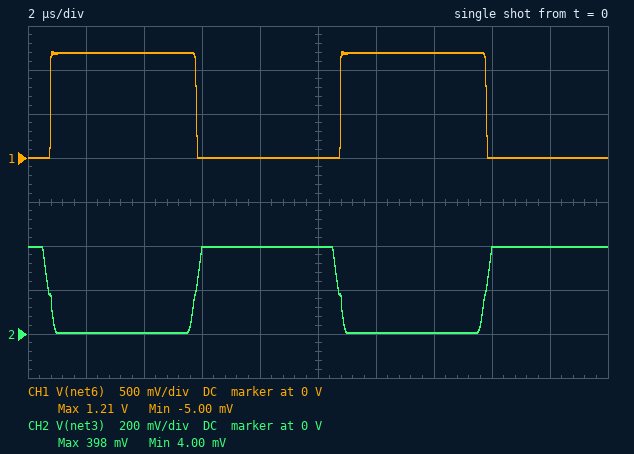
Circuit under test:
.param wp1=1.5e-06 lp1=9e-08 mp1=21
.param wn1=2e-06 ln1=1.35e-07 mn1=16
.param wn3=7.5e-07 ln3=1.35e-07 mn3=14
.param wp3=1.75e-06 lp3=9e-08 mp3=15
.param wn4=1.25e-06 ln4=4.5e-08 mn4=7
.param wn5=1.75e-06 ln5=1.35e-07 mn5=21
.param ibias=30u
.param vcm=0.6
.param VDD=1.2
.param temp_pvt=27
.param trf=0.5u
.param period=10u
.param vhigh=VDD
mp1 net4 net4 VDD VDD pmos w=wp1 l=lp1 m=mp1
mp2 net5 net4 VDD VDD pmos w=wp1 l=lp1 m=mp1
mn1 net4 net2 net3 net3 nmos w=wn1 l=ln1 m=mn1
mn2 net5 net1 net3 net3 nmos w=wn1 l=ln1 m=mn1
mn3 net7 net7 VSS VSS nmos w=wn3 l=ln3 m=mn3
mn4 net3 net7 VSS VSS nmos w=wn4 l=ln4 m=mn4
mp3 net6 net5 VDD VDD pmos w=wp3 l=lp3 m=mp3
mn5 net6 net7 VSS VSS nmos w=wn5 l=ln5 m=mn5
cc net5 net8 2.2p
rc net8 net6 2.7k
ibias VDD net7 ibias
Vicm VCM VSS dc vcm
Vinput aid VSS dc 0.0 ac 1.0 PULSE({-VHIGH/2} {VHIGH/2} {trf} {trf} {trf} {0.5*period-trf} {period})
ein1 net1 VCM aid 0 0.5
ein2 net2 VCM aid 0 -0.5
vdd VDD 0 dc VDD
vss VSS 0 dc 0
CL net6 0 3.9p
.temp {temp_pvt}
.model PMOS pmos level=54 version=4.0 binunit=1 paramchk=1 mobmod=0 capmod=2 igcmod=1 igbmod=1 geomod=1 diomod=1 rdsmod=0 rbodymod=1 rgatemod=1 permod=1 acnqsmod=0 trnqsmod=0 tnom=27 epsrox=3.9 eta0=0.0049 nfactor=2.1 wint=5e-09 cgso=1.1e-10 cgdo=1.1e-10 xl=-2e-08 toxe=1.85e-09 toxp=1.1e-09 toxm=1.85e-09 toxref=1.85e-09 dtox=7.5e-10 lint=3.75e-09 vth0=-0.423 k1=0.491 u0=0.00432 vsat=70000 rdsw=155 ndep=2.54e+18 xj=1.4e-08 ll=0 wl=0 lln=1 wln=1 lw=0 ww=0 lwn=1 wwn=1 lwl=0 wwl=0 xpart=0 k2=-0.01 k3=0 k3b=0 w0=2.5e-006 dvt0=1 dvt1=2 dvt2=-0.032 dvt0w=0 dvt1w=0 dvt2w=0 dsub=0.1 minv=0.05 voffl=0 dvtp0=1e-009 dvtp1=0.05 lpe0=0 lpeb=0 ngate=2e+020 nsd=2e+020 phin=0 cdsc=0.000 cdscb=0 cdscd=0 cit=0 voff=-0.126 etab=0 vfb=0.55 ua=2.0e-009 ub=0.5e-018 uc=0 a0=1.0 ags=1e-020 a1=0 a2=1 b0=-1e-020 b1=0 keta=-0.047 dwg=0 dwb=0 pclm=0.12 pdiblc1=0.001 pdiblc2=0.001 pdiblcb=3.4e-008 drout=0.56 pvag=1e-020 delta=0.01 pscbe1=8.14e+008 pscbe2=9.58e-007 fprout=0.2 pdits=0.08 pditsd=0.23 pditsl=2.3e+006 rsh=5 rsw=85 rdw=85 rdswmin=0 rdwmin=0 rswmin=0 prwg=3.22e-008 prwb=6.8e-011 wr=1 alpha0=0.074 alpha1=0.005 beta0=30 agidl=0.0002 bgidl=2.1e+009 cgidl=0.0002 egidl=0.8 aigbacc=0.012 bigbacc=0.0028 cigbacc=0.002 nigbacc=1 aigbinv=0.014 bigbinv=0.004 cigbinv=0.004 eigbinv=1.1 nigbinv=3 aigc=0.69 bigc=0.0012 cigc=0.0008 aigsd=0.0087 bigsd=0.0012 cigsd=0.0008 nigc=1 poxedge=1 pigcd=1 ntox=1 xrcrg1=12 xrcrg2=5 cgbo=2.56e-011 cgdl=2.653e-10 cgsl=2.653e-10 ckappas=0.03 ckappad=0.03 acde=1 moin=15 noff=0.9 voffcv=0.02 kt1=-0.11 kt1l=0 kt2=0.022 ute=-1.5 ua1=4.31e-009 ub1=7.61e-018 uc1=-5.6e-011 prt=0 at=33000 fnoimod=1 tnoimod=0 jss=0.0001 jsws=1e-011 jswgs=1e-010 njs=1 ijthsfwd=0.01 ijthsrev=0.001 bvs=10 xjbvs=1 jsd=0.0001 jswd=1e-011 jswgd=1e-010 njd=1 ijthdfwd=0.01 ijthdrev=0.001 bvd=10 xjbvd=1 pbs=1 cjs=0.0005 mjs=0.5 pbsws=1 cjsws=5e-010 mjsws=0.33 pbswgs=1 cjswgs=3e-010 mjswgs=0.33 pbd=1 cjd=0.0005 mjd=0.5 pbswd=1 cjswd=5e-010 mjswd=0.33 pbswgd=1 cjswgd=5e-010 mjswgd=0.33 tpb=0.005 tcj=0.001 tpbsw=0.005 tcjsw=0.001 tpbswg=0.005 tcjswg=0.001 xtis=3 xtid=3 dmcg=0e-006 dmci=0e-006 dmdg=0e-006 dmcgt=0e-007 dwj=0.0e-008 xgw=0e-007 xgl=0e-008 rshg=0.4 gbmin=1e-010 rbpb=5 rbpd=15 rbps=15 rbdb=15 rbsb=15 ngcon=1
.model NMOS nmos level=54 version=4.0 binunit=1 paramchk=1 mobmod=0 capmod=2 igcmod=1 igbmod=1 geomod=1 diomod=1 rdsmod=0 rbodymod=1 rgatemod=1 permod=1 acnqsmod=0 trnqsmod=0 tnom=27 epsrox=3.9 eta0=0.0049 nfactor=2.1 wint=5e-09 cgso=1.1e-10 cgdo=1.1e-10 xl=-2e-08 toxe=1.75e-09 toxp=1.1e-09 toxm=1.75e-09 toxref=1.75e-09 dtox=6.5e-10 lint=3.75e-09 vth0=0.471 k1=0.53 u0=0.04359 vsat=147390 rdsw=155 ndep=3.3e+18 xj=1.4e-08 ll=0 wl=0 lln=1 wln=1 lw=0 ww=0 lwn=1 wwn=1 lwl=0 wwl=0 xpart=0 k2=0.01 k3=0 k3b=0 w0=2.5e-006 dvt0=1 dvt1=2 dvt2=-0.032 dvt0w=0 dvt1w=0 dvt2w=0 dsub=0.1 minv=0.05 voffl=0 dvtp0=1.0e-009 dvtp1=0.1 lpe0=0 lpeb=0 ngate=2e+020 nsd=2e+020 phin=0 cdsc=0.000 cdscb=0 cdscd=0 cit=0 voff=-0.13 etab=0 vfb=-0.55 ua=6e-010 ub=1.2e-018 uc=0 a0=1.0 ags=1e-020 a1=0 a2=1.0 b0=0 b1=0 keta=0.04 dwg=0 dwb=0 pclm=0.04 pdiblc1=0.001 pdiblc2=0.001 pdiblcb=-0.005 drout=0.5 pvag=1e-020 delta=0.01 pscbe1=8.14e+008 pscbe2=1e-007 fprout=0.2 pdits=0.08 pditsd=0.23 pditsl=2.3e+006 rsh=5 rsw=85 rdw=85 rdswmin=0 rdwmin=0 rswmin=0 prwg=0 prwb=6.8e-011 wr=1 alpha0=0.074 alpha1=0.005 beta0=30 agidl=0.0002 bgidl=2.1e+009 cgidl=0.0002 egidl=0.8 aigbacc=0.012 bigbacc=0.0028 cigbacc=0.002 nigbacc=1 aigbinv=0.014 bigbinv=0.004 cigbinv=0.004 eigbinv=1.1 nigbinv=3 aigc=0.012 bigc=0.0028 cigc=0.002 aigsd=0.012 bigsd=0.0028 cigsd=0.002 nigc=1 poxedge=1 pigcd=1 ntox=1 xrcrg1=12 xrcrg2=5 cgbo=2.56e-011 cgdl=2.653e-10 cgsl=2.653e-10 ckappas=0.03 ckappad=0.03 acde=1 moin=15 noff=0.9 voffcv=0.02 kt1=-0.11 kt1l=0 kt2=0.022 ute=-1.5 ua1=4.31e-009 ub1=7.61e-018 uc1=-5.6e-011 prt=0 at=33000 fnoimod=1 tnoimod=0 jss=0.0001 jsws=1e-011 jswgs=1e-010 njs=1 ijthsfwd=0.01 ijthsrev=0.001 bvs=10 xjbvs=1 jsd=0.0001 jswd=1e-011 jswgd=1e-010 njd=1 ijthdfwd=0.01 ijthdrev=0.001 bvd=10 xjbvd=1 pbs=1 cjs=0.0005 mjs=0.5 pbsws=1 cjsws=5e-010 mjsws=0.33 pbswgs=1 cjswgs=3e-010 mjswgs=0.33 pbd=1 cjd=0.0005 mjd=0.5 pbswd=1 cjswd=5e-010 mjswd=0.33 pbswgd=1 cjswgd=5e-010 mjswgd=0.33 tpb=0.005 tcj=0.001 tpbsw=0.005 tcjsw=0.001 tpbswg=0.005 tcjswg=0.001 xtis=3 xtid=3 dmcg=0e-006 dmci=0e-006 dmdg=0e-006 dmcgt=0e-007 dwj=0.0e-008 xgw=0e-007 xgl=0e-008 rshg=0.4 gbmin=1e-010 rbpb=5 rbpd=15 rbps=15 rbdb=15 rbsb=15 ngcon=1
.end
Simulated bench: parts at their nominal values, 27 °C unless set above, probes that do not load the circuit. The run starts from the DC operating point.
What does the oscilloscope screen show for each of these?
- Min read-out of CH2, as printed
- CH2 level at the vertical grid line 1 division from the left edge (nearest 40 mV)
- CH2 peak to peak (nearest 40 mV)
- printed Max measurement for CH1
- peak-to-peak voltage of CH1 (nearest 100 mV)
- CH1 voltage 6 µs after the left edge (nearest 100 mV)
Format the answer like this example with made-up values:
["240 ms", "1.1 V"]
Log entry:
["4.00 mV", "0 V", "400 mV", "1.21 V", "1.2 V", "0 V"]
